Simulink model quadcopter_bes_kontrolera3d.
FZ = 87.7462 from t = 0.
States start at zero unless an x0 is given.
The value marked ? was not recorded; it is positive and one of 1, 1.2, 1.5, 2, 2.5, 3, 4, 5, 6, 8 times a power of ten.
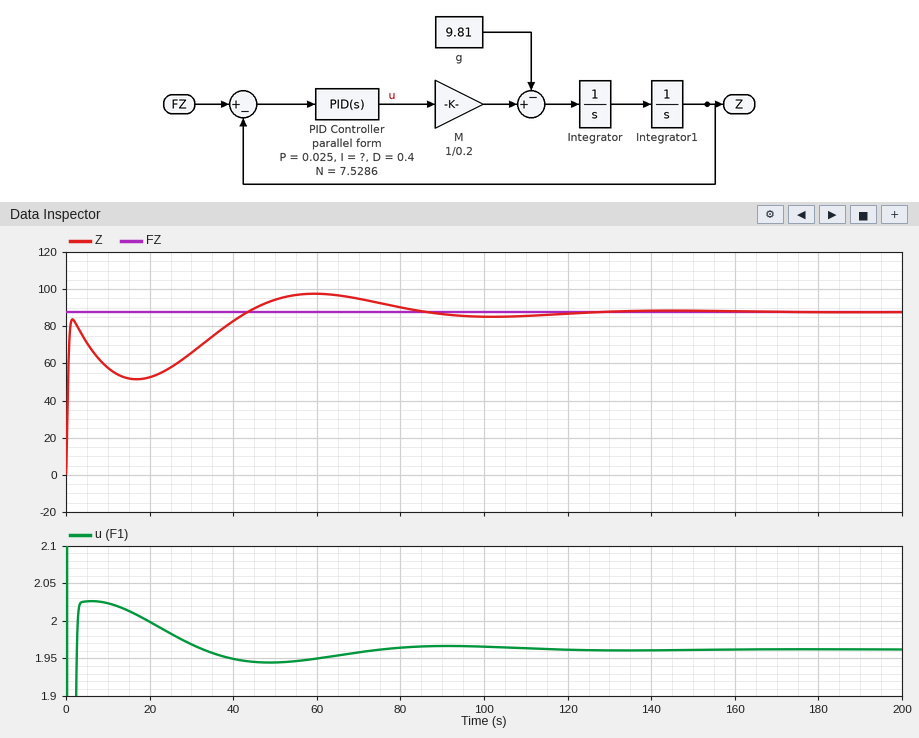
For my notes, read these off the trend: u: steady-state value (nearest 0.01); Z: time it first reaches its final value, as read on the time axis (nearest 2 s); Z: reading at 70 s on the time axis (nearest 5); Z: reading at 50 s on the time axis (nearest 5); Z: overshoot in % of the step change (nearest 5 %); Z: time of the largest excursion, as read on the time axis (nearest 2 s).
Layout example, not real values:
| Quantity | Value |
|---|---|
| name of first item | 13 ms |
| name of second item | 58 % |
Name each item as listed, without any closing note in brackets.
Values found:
| Quantity | Value |
|---|---|
| u: steady-state value | 1.96 |
| Z: time it first reaches its final value, as read on the time axis | 44 s |
| Z: reading at 70 s on the time axis | 95 |
| Z: reading at 50 s on the time axis | 95 |
| Z: overshoot in % of the step change | 10 % |
| Z: time of the largest excursion, as read on the time axis | 60 s |
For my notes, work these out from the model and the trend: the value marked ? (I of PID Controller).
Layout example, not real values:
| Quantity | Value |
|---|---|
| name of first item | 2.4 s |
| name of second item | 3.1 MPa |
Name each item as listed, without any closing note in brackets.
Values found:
| Quantity | Value |
|---|---|
| the value marked ? | 0.0025 |
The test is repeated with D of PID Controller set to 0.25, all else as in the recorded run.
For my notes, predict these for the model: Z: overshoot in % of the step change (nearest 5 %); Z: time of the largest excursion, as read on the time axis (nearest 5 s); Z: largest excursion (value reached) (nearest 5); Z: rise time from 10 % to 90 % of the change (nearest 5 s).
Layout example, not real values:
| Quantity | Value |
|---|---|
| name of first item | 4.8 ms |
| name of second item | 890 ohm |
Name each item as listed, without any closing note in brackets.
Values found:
| Quantity | Value |
|---|---|
| Z: overshoot in % of the step change | 10 % |
| Z: time of the largest excursion, as read on the time axis | 50 s |
| Z: largest excursion (value reached) | 95 |
| Z: rise time from 10 % to 90 % of the change | 30 s |
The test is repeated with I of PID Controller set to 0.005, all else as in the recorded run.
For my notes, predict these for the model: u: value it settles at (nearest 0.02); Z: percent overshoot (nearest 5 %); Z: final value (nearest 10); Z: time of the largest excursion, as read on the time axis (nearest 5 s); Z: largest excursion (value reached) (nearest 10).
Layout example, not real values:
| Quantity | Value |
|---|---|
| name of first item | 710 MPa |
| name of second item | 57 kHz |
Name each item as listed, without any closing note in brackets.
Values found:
| Quantity | Value |
|---|---|
| u: value it settles at | 1.96 |
| Z: percent overshoot | 15 % |
| Z: final value | 90 |
| Z: time of the largest excursion, as read on the time axis | 40 s |
| Z: largest excursion (value reached) | 100 |
